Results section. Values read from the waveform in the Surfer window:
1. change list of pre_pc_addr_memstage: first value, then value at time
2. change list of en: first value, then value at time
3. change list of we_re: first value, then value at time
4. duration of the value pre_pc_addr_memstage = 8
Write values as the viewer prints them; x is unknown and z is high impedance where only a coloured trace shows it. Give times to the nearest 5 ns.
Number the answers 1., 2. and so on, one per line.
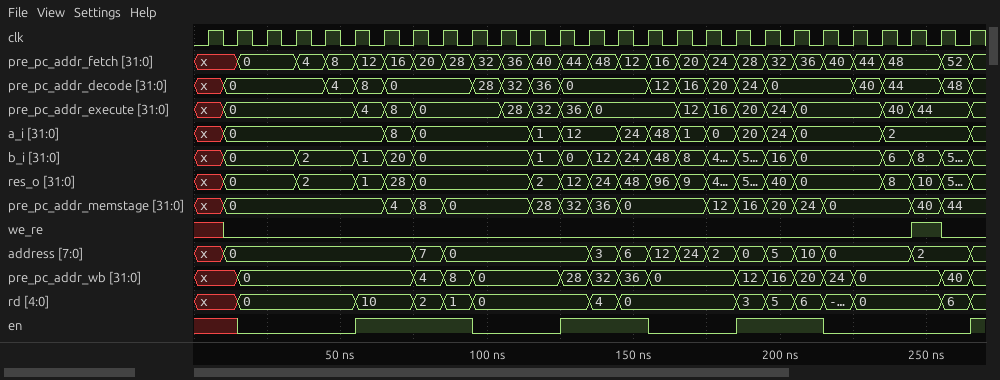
1. x, 0 at 10 ns, 4 at 65 ns, 8 at 75 ns, 0 at 85 ns, 28 at 115 ns, 32 at 125 ns, 36 at 135 ns, 0 at 145 ns, 12 at 175 ns, 16 at 185 ns, 20 at 195 ns, 24 at 205 ns, 0 at 215 ns, 40 at 245 ns, 44 at 255 ns
2. x, 0 at 15 ns, 1 at 55 ns, 0 at 95 ns, 1 at 125 ns, 0 at 155 ns, 1 at 185 ns, 0 at 215 ns, 1 at 265 ns
3. x, 0 at 10 ns, 1 at 245 ns, 0 at 255 ns
4. 10 ns
